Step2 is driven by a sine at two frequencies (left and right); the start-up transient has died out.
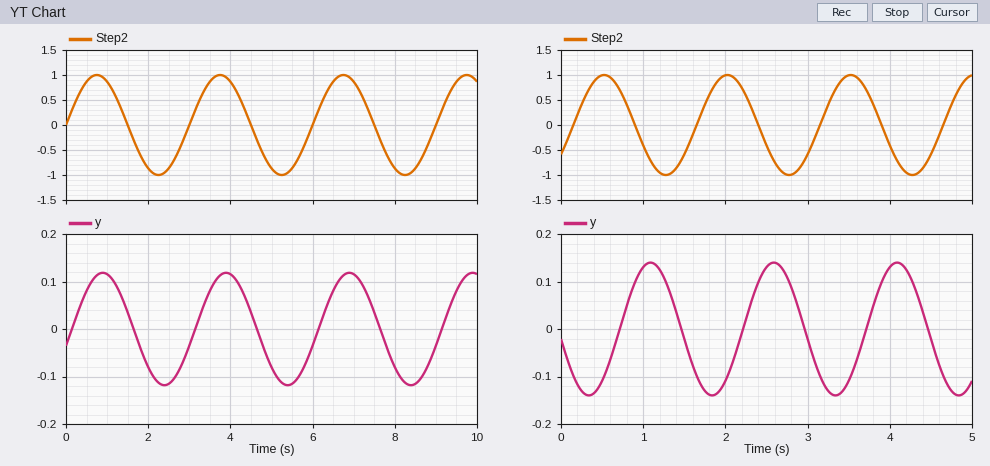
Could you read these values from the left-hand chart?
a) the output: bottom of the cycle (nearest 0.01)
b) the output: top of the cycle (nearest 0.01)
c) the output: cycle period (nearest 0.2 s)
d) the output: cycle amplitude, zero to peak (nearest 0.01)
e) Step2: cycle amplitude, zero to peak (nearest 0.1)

-0.12
0.12
3.0 s
0.12
1.0
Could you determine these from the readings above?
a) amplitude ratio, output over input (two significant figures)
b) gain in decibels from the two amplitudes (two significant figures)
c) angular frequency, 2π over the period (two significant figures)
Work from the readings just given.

0.12
-18 dB
2.1 rad/s
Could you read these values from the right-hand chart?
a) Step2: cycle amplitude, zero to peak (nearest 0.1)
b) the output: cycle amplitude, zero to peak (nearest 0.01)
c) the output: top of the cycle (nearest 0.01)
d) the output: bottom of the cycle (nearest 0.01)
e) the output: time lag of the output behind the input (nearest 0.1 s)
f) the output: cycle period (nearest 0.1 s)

1.0
0.14
0.14
-0.14
0.6 s
1.5 s
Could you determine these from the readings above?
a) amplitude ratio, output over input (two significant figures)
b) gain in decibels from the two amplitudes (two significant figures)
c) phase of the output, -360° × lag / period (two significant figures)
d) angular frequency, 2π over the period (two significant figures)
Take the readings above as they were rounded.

0.14
-17 dB
-140°
4.2 rad/s
